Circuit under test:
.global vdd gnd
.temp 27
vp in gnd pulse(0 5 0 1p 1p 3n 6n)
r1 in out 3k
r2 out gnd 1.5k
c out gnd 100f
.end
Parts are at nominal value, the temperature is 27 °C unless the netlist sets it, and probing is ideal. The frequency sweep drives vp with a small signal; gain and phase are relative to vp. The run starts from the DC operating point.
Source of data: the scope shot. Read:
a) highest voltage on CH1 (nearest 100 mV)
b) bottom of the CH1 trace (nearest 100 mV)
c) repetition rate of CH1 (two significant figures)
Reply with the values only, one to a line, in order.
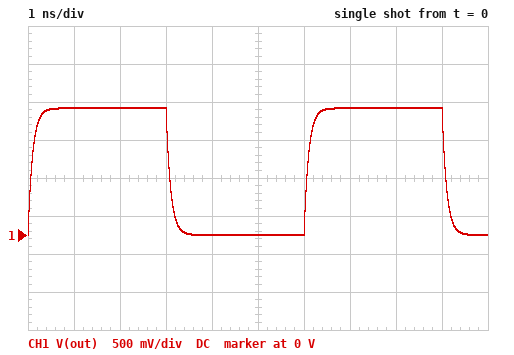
1.7 V
0 V
170 MHz
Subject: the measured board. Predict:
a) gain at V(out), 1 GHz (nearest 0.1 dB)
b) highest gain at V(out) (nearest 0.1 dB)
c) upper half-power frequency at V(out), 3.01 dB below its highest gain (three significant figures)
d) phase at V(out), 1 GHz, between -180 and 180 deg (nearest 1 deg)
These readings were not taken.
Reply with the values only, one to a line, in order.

-11.0 dB
-9.5 dB
1.59 GHz
-32 deg
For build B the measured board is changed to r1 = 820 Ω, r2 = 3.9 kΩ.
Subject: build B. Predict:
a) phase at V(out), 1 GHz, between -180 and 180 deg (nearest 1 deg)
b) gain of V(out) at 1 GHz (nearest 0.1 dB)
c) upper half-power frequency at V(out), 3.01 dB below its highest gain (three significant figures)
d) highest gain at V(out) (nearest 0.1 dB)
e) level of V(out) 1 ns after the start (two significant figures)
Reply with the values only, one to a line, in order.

-23 deg
-2.4 dB
2.35 GHz
-1.7 dB
4.1 V
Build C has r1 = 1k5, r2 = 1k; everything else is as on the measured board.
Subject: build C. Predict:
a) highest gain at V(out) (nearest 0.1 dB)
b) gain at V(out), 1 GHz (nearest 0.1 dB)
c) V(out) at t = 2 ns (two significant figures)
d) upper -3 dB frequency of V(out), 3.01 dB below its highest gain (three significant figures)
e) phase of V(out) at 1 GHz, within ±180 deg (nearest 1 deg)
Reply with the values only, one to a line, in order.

-8.0 dB
-8.5 dB
2.0 V
2.65 GHz
-21 deg
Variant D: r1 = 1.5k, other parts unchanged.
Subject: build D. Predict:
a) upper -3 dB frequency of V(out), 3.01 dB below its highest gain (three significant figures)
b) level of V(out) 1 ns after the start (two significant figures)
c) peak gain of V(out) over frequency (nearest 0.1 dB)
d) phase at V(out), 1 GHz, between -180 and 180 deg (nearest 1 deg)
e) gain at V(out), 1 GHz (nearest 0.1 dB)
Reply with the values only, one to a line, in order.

2.12 GHz
2.5 V
-6.0 dB
-25 deg
-6.9 dB
